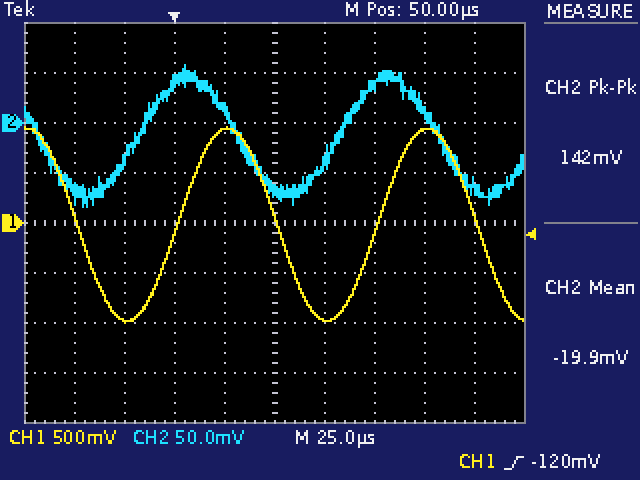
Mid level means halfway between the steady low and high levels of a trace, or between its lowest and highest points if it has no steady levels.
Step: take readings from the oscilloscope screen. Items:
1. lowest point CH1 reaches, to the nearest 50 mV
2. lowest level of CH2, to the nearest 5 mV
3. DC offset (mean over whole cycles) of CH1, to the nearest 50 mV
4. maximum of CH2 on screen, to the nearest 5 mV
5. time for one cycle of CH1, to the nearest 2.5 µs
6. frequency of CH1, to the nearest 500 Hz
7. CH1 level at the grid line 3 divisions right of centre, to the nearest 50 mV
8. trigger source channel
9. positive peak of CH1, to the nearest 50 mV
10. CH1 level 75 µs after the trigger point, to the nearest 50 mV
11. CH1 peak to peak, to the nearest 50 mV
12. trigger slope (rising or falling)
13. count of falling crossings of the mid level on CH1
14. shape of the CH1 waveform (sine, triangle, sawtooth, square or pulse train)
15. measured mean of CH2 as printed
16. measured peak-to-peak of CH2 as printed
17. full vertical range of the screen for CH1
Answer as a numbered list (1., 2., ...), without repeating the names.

1. -1.00 V
2. -85 mV
3. 0 mV
4. 60 mV
5. 100.0 µs
6. 10.0 kHz
7. 950 mV
8. CH1
9. 950 mV
10. -950 mV
11. 1.95 V
12. rising
13. 3
14. sine
15. -19.9 mV
16. 142 mV
17. 4 V
